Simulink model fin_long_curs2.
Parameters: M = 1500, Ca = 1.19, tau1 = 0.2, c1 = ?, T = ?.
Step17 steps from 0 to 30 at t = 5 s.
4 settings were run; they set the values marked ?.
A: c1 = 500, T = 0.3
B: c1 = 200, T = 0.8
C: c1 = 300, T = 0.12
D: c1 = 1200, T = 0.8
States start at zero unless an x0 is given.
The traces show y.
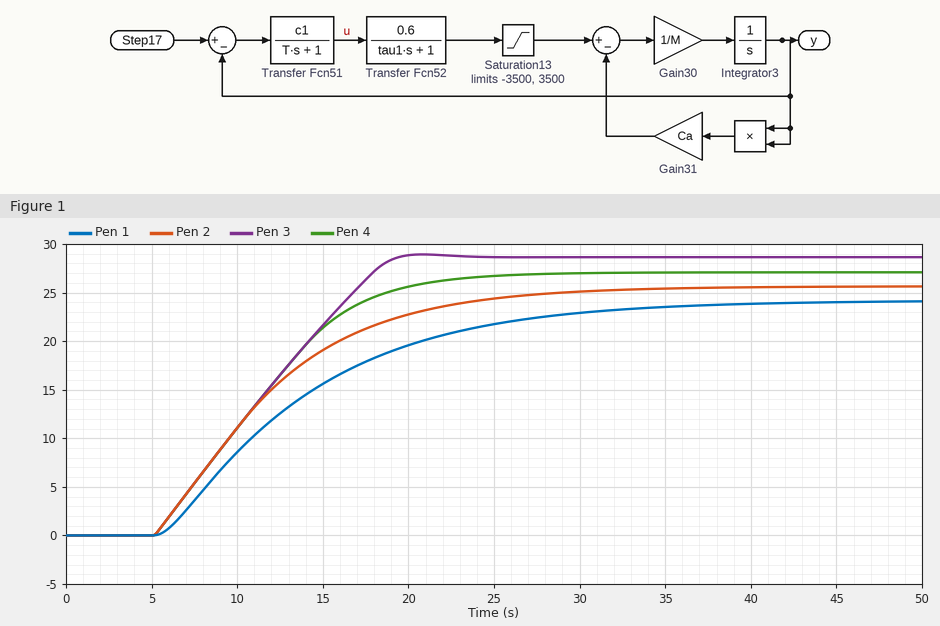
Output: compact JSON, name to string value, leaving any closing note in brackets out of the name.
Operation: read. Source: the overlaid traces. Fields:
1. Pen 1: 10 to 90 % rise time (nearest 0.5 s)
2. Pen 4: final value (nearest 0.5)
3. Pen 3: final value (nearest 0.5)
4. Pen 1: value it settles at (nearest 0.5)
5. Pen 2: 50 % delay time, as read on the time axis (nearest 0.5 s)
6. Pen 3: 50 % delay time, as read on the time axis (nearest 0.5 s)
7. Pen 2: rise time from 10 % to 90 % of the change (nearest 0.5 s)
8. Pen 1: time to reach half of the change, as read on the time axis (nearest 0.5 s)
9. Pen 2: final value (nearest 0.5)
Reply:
{"Pen 1: 10 to 90 % rise time": "18.0 s", "Pen 4: final value": "27.0", "Pen 3: final value": "28.5", "Pen 1: value it settles at": "24.0", "Pen 2: 50 % delay time, as read on the time axis": "11.0 s", "Pen 3: 50 % delay time, as read on the time axis": "11.5 s", "Pen 2: rise time from 10 % to 90 % of the change": "14.5 s", "Pen 1: time to reach half of the change, as read on the time axis": "12.0 s", "Pen 2: final value": "25.5"}
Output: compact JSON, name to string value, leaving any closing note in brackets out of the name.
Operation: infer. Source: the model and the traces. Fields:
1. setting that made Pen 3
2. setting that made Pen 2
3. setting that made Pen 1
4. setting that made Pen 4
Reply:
{"setting that made Pen 3": "D", "setting that made Pen 2": "C", "setting that made Pen 1": "B", "setting that made Pen 4": "A"}
